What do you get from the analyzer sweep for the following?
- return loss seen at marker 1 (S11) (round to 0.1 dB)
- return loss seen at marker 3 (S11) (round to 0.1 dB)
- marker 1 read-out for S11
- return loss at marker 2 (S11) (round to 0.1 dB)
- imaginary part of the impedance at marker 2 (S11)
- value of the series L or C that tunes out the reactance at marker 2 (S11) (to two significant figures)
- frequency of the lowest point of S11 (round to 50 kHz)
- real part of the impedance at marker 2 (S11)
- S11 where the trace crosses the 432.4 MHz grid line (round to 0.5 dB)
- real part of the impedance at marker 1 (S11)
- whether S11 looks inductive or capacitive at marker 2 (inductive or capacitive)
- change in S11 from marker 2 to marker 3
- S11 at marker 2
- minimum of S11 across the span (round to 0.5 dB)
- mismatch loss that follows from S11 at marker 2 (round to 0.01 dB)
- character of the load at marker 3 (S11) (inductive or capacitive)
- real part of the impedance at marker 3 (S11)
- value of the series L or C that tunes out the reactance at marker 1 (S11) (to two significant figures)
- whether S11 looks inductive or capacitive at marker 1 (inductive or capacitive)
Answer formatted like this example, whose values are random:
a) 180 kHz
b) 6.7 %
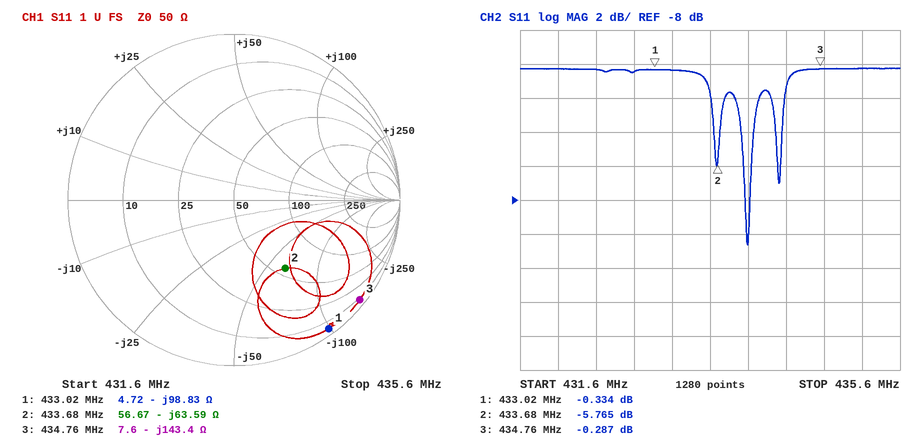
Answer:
a) 0.3 dB
b) 0.3 dB
c) -0.334 dB
d) 5.8 dB
e) -63.59 Ω
f) 23 nH
g) 434.00 MHz
h) 56.67 Ω
i) -0.5 dB
j) 4.72 Ω
k) capacitive
l) 5.478 dB
m) -5.765 dB
n) -10.5 dB
o) 1.34 dB
p) capacitive
q) 7.6 Ω
r) 36 nH
s) capacitive
